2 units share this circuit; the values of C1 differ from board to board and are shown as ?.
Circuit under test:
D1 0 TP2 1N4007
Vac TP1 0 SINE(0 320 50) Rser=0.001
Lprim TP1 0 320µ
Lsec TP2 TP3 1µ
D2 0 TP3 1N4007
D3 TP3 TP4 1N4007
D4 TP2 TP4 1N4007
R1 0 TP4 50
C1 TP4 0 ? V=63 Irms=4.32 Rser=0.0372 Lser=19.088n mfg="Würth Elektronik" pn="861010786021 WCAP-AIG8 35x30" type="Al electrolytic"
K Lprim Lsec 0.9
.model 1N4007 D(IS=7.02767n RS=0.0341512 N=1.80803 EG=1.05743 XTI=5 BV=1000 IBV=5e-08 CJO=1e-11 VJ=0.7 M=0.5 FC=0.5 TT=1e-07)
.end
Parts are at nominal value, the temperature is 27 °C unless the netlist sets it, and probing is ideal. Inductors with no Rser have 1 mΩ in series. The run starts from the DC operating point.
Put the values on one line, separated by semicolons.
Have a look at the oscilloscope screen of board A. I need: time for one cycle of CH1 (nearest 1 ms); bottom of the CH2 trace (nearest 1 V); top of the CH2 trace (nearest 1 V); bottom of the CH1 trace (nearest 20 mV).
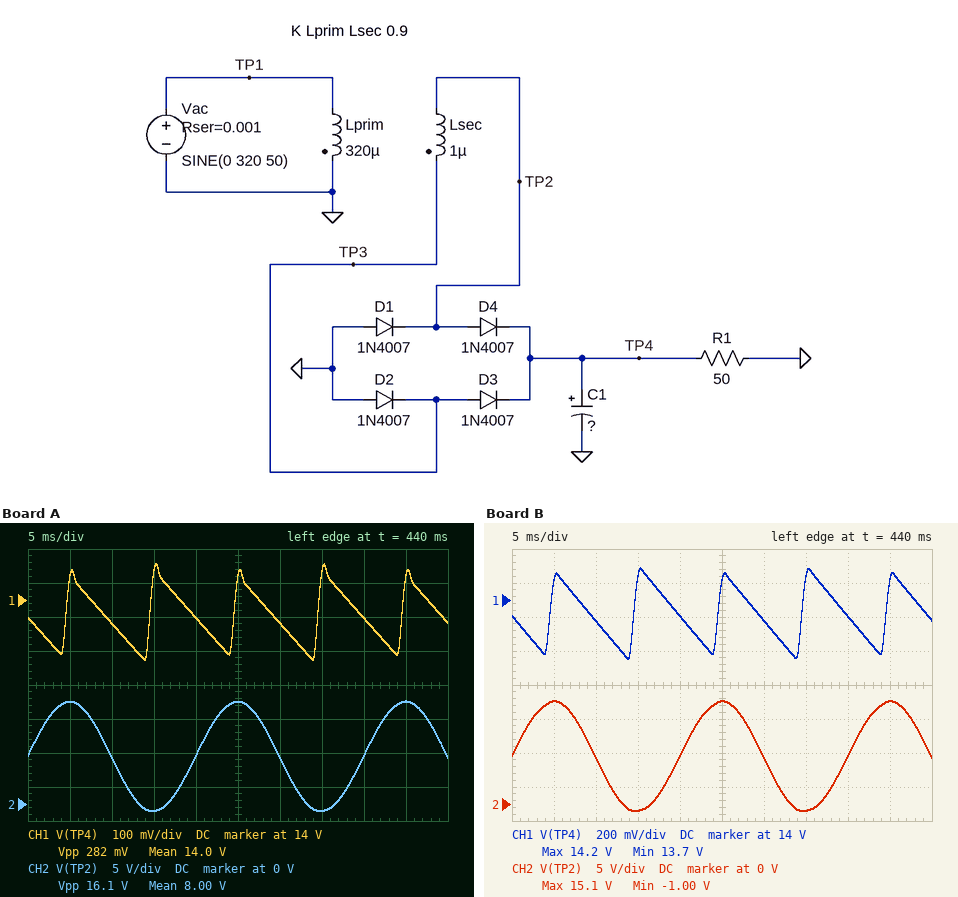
10 ms; -1 V; 15 V; 13.82 V
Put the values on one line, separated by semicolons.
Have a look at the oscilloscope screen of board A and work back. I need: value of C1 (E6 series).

10 mF
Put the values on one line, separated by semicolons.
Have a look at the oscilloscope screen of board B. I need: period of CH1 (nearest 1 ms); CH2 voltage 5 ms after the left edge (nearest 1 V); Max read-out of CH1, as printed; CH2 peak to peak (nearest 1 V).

10 ms; 15 V; 14.2 V; 16 V
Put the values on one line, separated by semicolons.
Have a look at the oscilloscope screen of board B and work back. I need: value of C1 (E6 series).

4.7 mF
